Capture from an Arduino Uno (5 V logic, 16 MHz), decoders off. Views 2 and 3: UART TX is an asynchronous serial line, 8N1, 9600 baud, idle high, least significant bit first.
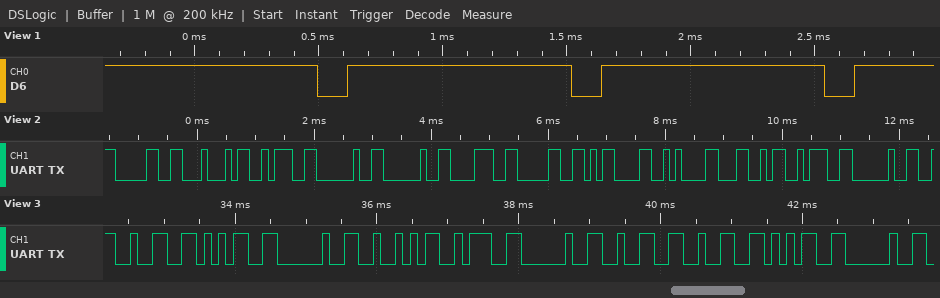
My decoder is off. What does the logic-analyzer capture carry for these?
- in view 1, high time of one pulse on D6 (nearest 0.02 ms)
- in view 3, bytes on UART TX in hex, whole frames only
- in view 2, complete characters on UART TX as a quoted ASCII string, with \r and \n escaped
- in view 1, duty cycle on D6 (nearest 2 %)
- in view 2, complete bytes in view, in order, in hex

0.90 ms
32 35 20 52 3A 20 32 32 35 20
"0D:  80\r\nL: "
88 %
30 44 3A 20 20 38 30 0D 0A 4C 3A 20
